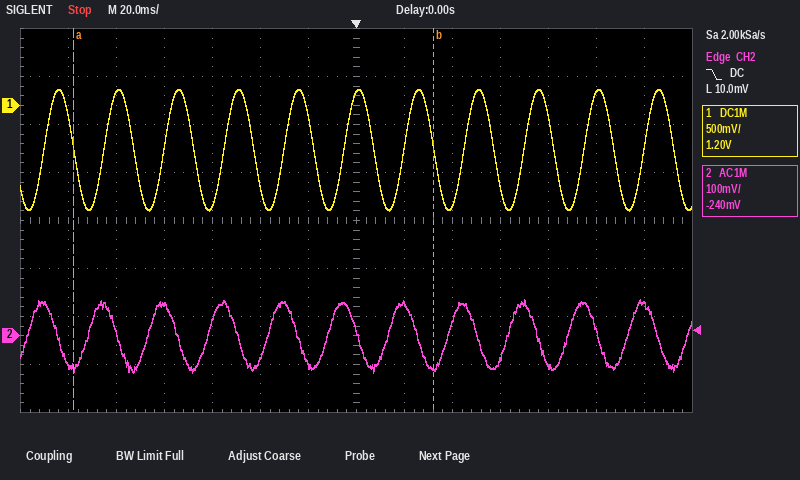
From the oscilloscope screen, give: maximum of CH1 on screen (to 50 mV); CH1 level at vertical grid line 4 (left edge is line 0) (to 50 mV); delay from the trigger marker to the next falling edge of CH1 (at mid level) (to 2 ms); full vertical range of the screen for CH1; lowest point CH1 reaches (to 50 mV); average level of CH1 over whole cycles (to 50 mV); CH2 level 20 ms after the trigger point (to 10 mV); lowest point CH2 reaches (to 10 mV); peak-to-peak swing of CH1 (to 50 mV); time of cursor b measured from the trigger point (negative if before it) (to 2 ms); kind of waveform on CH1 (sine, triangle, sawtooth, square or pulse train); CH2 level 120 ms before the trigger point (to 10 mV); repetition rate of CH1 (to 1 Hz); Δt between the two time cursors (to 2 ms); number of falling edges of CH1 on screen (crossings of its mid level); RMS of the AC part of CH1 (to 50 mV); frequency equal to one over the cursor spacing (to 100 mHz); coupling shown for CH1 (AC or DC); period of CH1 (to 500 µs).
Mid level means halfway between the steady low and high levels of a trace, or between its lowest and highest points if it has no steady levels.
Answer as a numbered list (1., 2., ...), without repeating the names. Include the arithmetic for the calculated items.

1. 150 mV
2. -1.05 V
3. 8 ms
4. 4 V
5. -1.10 V
6. (150 mV + (-1.10 V)) / 2 ≈ -475 mV, so -450 mV to the nearest 50 mV
7. 70 mV
8. -80 mV
9. 150 mV − (-1.10 V) = 1.25 V
10. +32 ms
11. sine
12. -60 mV
13. 1 / 25.0 ms ≈ 40 Hz
14. 150 ms
15. 11
16. 1.25 V / (2√2) ≈ 442 mV, so 450 mV to the nearest 50 mV
17. 1 / 150 ms ≈ 6.7 Hz
18. DC
19. 25.0 ms
